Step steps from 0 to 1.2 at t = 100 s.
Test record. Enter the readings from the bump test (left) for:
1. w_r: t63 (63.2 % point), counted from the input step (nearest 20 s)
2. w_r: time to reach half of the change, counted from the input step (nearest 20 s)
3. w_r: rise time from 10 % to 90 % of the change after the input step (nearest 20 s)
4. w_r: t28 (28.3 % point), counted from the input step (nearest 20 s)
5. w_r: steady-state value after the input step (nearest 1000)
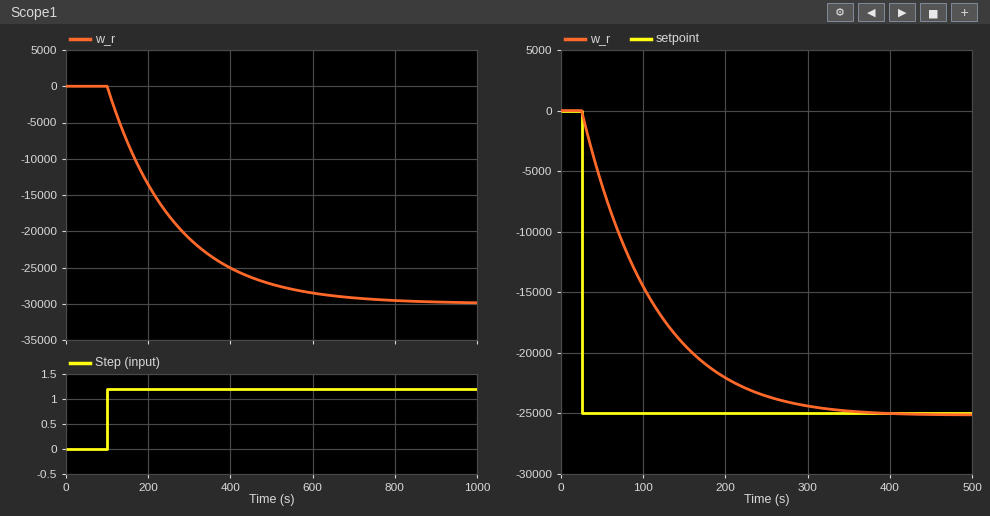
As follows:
160 s
120 s
360 s
60 s
-30000
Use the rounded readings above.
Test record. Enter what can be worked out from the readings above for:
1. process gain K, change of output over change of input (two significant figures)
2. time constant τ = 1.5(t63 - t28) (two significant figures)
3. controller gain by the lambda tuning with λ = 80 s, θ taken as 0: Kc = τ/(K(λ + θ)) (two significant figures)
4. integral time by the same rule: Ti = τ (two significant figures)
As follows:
-25000
150 s
-0.000075
150 s
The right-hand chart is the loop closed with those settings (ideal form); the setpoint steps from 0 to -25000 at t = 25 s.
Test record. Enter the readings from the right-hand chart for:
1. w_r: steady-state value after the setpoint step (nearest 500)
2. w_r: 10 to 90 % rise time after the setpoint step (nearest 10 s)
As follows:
-25000
180 s
